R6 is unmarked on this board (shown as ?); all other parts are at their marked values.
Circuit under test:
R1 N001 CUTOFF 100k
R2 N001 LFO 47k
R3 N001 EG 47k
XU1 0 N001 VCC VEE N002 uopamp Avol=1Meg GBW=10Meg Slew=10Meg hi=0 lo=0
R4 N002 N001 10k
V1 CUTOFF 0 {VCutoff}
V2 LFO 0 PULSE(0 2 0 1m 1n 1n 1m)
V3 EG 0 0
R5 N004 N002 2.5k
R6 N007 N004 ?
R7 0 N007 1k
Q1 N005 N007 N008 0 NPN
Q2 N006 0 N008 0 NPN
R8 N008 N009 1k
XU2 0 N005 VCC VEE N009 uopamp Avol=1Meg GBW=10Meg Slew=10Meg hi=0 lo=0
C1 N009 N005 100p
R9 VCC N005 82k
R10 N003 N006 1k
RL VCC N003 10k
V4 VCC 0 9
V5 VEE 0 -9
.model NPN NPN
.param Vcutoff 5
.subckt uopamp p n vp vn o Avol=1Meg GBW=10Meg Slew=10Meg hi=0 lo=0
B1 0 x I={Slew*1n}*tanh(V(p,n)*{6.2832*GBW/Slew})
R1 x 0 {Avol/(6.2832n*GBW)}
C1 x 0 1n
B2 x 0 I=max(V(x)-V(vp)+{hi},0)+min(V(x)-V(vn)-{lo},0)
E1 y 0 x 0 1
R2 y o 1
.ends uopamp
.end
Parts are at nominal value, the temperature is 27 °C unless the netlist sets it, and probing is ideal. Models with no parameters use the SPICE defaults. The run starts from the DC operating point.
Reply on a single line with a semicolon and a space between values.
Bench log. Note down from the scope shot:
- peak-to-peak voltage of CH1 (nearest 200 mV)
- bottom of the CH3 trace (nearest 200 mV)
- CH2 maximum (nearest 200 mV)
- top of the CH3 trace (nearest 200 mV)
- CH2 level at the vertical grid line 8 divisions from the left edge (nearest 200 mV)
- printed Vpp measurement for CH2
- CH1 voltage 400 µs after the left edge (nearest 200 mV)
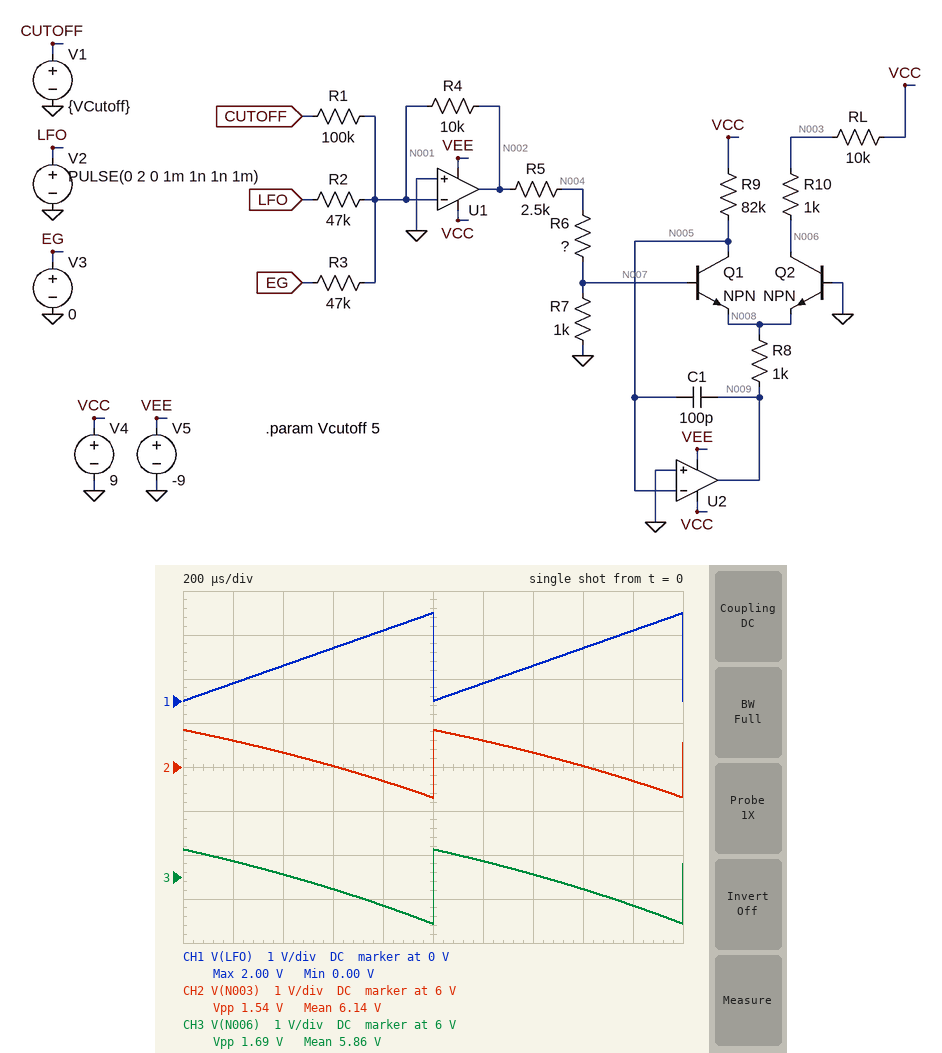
2.0 V; 5.0 V; 6.8 V; 6.6 V; 6.0 V; 1.54 V; 800 mV
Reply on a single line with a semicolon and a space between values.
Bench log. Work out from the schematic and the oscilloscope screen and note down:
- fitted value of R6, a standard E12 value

27 kΩ
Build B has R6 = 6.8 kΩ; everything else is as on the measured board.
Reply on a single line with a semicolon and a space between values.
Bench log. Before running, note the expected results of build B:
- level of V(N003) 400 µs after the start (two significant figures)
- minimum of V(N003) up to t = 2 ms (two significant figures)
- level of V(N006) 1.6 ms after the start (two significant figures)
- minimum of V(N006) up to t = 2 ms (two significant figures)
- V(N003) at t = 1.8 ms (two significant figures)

150 mV; 110 mV; -760 mV; -780 mV; 120 mV
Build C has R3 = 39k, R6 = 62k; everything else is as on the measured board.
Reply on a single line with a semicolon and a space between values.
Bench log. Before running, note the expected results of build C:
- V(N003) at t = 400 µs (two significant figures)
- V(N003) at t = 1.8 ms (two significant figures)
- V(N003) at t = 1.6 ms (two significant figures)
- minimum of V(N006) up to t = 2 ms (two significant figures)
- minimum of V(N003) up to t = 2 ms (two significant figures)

7.3 V; 7.1 V; 7.2 V; 6.8 V; 7.0 V
